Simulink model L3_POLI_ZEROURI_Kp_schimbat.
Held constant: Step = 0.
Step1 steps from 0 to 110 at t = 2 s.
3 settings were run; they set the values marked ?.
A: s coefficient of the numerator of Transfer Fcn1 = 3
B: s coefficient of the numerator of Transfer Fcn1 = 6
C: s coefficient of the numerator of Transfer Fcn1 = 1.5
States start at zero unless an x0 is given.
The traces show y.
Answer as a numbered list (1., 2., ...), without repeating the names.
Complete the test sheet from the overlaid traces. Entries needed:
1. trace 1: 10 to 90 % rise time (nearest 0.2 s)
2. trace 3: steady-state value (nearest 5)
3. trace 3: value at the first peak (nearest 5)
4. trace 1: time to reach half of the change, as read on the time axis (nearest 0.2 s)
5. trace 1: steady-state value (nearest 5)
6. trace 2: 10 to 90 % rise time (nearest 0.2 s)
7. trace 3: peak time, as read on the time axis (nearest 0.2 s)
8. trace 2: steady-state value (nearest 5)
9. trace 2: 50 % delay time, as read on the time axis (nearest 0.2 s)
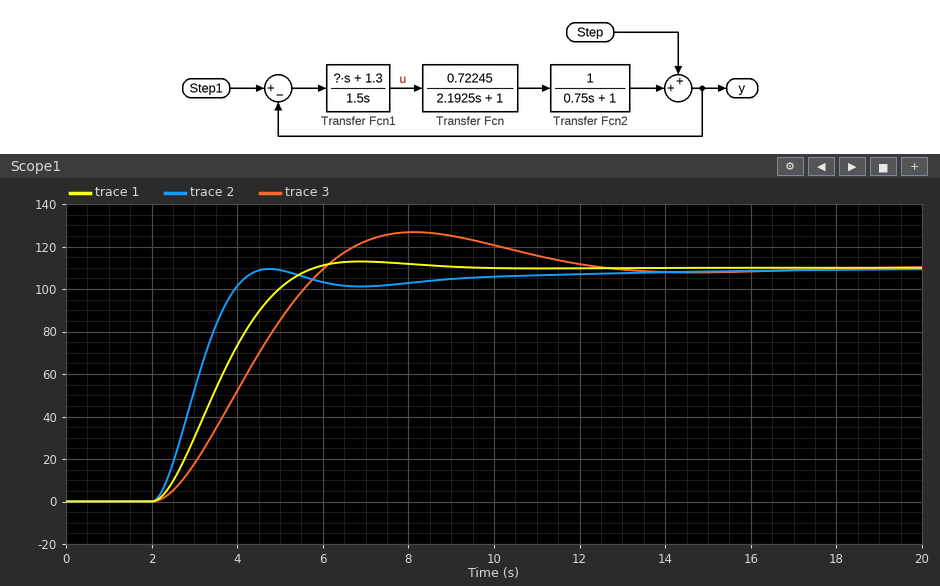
1. 2.4 s
2. 110
3. 125
4. 3.6 s
5. 110
6. 1.6 s
7. 8.2 s
8. 110
9. 3.0 s
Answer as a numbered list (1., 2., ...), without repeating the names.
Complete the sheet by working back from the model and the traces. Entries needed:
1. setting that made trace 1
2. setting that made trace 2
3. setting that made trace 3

1. A
2. B
3. C
